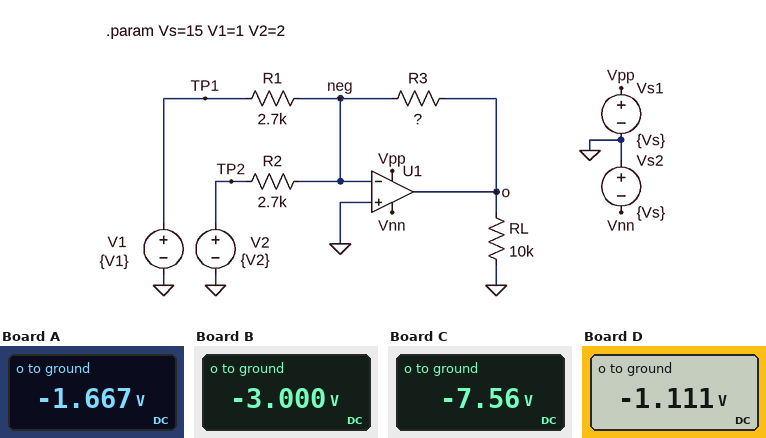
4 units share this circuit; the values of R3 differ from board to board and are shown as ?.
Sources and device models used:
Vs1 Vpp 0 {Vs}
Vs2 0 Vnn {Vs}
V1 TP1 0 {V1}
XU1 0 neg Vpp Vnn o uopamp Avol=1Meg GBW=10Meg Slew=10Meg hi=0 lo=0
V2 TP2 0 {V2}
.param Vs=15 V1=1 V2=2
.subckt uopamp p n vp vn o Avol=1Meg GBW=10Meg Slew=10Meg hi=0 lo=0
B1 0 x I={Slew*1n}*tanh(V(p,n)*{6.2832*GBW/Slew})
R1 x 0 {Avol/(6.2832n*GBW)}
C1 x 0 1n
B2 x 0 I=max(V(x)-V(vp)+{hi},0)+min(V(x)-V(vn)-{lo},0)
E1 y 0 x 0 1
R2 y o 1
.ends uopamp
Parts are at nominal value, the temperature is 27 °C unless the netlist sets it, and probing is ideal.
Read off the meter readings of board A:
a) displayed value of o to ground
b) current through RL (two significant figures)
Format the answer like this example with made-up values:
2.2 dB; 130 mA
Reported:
-1.667 V; 170 µA
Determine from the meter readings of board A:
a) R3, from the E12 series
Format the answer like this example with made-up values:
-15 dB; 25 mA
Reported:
1.5 kΩ
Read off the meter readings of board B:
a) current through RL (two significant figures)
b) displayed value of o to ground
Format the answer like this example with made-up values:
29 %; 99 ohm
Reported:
300 µA; -3.000 V
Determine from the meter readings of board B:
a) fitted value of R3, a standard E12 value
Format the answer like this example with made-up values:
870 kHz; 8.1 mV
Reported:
2.7 kΩ
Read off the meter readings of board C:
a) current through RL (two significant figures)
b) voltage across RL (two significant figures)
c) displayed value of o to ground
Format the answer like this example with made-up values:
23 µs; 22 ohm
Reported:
760 µA; 7.6 V; -7.56 V
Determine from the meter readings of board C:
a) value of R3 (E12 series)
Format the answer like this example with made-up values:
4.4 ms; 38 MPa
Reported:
6.8 kΩ
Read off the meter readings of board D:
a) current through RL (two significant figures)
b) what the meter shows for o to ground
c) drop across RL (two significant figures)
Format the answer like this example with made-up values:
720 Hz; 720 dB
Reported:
110 µA; -1.111 V; 1.1 V
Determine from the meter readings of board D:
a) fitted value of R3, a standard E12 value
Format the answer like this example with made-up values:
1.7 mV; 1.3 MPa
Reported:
1 kΩ
